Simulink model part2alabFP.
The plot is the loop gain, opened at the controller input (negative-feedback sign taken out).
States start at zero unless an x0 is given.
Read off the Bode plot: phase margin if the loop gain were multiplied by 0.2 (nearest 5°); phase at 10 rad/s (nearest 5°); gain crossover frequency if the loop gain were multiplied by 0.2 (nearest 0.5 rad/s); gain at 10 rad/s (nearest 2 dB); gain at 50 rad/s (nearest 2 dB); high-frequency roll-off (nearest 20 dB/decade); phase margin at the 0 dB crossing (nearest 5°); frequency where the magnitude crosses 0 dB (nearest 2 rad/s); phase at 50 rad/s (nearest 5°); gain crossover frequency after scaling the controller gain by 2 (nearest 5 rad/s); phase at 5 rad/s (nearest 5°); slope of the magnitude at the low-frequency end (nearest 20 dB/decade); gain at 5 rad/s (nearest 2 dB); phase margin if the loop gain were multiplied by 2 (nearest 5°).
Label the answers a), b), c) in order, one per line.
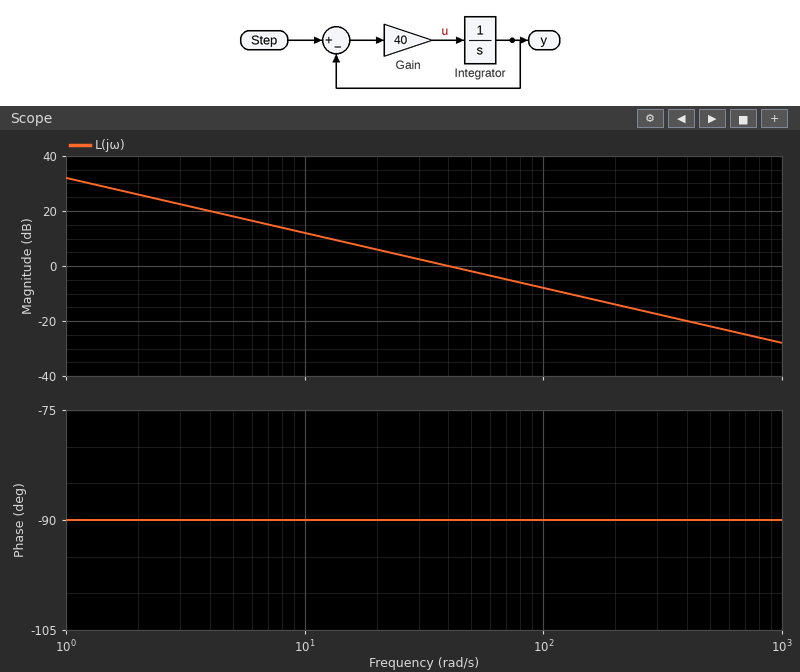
a) 90°
b) -90°
c) 8.0 rad/s
d) 12 dB
e) -2 dB
f) -20 dB/decade
g) 90°
h) 40 rad/s
i) -90°
j) 80 rad/s
k) -90°
l) -20 dB/decade
m) 18 dB
n) 90°
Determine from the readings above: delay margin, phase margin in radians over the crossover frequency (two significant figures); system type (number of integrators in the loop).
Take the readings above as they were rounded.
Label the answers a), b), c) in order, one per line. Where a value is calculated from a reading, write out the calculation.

a) 90 × π / 180 / 40 = 0.039 s
b) 1
